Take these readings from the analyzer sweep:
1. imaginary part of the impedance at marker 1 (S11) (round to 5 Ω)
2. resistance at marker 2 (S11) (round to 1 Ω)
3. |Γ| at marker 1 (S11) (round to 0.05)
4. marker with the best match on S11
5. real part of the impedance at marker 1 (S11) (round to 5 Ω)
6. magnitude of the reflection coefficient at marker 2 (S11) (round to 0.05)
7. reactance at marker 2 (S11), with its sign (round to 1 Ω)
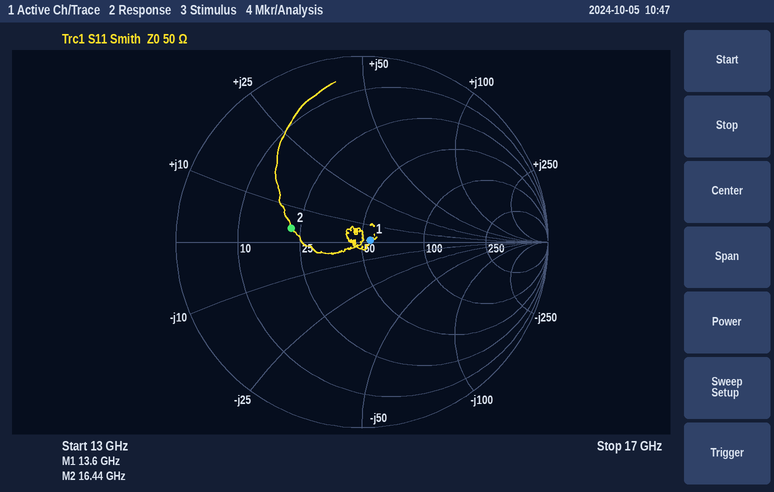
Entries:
0 Ω
22 Ω
0.05
marker 1
55 Ω
0.40
+4 Ω
